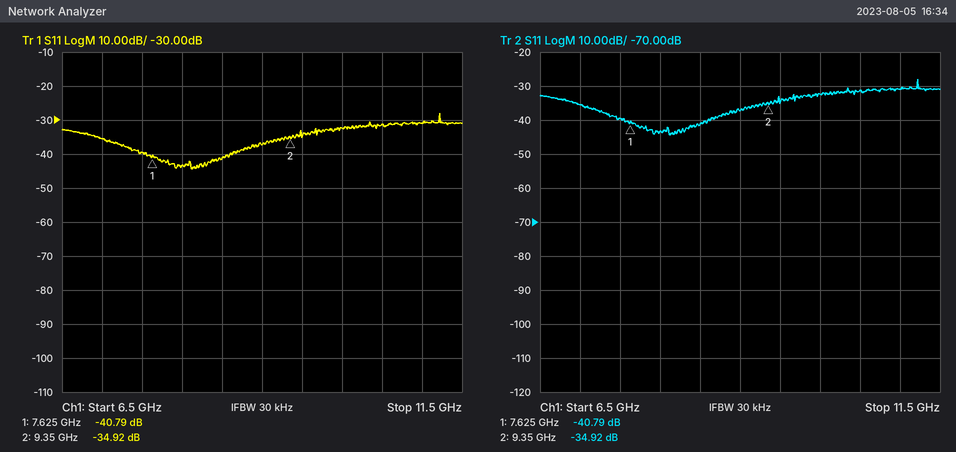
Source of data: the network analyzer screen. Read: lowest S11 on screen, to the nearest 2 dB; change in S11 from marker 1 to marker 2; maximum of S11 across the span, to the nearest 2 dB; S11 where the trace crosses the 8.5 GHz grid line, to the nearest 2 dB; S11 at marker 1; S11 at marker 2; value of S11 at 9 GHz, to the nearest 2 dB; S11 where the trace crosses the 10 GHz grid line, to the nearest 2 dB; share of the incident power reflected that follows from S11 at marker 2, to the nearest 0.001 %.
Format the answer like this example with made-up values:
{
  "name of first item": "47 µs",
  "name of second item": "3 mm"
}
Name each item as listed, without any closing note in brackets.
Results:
{
  "lowest S11 on screen, to the nearest 2 dB": "-44 dB",
  "change in S11 from marker 1 to marker 2": "5.87 dB",
  "maximum of S11 across the span, to the nearest 2 dB": "-28 dB",
  "S11 where the trace crosses the 8.5 GHz grid line, to the nearest 2 dB": "-42 dB",
  "S11 at marker 1": "-40.79 dB",
  "S11 at marker 2": "-34.92 dB",
  "value of S11 at 9 GHz, to the nearest 2 dB": "-38 dB",
  "S11 where the trace crosses the 10 GHz grid line, to the nearest 2 dB": "-32 dB",
  "share of the incident power reflected that follows from S11 at marker 2, to the nearest 0.001 %": "0.032 %"
}
